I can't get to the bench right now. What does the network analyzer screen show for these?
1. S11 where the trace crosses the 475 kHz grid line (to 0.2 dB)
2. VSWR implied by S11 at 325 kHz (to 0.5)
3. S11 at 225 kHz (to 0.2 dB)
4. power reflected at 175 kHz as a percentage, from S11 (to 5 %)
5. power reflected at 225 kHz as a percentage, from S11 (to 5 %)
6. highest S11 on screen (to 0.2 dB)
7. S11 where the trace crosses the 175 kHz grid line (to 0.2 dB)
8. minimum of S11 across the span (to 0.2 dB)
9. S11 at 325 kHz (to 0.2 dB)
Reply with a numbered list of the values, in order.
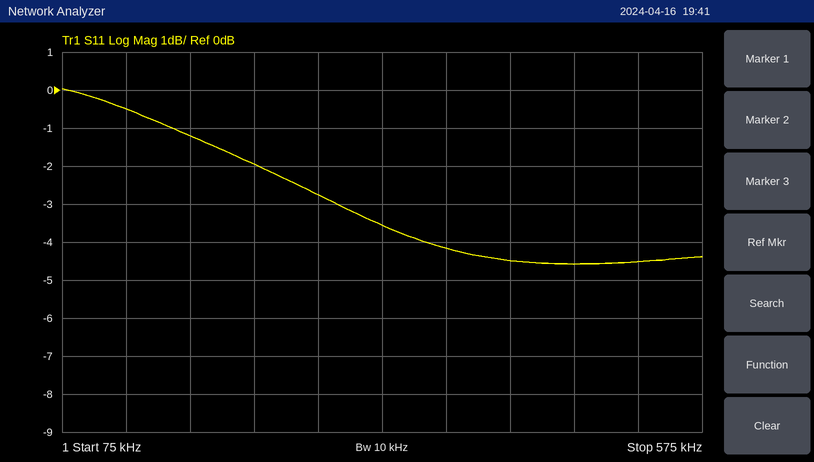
1. -4.6 dB
2. 5.0
3. -2.0 dB
4. 75 %
5. 65 %
6. 0.0 dB
7. -1.2 dB
8. -4.6 dB
9. -3.6 dB
